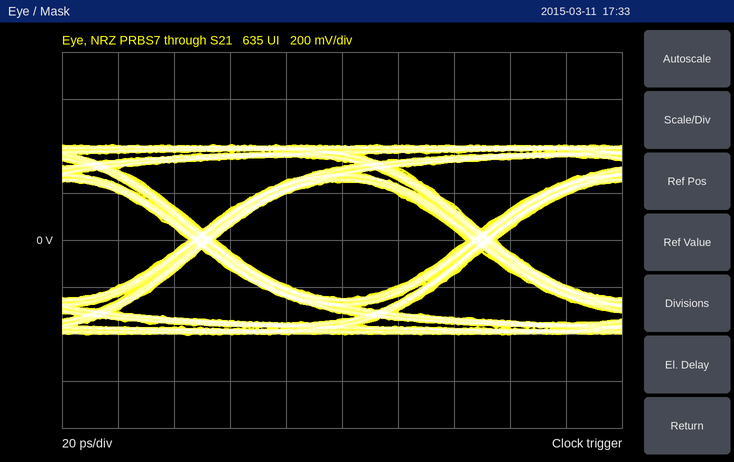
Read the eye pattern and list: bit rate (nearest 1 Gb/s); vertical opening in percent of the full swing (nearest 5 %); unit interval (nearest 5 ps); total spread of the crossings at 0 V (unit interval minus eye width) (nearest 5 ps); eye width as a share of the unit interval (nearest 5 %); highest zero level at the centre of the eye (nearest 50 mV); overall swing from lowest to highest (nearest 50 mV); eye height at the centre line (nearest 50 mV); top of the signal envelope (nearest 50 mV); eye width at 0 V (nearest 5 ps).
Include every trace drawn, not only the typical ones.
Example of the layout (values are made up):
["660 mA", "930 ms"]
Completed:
["10 Gb/s", "60 %", "100 ps", "10 ps", "90 %", "-250 mV", "800 mV", "500 mV", "400 mV", "90 ps"]
